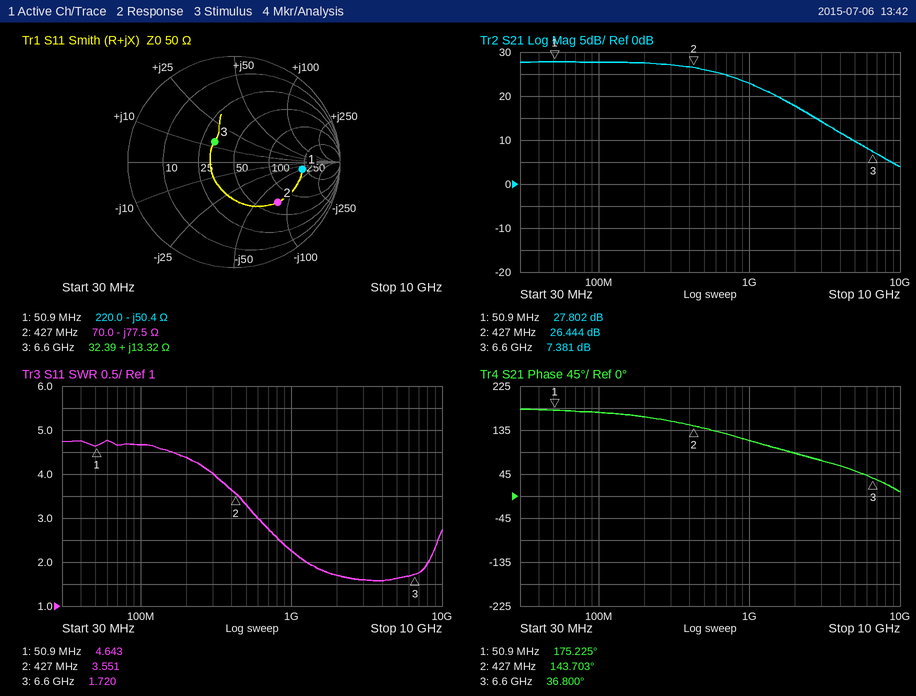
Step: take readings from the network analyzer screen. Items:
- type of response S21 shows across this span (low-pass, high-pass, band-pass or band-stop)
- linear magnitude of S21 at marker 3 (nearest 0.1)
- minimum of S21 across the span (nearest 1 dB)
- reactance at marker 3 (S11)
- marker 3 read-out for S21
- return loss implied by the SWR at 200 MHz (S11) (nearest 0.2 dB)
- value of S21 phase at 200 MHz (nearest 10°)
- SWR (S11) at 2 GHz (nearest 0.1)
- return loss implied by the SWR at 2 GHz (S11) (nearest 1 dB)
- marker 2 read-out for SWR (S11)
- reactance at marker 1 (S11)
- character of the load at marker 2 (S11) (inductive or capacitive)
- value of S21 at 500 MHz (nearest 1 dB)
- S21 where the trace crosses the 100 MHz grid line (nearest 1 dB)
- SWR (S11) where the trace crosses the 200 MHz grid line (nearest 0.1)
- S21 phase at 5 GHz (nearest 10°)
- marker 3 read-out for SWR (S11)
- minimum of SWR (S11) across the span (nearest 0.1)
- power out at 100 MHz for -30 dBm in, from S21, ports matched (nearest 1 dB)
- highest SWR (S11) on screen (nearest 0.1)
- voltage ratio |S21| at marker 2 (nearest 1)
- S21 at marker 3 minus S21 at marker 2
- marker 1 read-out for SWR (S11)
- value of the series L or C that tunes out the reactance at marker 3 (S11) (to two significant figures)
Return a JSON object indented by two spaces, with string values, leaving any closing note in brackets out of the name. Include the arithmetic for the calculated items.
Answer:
{
  "type of response S21 shows across this span": "low-pass",
  "linear magnitude of S21 at marker 3": "10^(7.381/20) ≈ 2.3",
  "minimum of S21 across the span": "4 dB",
  "reactance at marker 3": "+13.32 Ω",
  "marker 3 read-out for S21": "7.381 dB",
  "return loss implied by the SWR at 200 MHz (S11)": "−20 log10((4.4 − 1)/(4.4 + 1)) ≈ 4.0 dB",
  "value of S21 phase at 200 MHz": "160°",
  "SWR (S11) at 2 GHz": "1.7",
  "return loss implied by the SWR at 2 GHz (S11)": "−20 log10((1.7 − 1)/(1.7 + 1)) ≈ 12 dB",
  "marker 2 read-out for SWR": "3.551",
  "reactance at marker 1": "-50.4 Ω",
  "character of the load at marker 2 (S11)": "capacitive",
  "value of S21 at 500 MHz": "26 dB",
  "S21 where the trace crosses the 100 MHz grid line": "28 dB",
  "SWR (S11) where the trace crosses the 200 MHz grid line": "4.4",
  "S21 phase at 5 GHz": "50°",
  "marker 3 read-out for SWR": "1.720",
  "minimum of SWR (S11) across the span": "1.6",
  "power out at 100 MHz for -30 dBm in, from S21, ports matched": "-30 dBm + (28 dB) = -2 dBm",
  "highest SWR (S11) on screen": "4.8",
  "voltage ratio |S21| at marker 2": "10^(26.444/20) ≈ 21",
  "S21 at marker 3 minus S21 at marker 2": "7.381 − (26.444) = -19.063 dB",
  "marker 1 read-out for SWR": "4.643",
  "value of the series L or C that tunes out the reactance at marker 3 (S11)": "C = 1/(2π × 6.6 GHz × 13.32 Ω) ≈ 1.8 pF"
}
